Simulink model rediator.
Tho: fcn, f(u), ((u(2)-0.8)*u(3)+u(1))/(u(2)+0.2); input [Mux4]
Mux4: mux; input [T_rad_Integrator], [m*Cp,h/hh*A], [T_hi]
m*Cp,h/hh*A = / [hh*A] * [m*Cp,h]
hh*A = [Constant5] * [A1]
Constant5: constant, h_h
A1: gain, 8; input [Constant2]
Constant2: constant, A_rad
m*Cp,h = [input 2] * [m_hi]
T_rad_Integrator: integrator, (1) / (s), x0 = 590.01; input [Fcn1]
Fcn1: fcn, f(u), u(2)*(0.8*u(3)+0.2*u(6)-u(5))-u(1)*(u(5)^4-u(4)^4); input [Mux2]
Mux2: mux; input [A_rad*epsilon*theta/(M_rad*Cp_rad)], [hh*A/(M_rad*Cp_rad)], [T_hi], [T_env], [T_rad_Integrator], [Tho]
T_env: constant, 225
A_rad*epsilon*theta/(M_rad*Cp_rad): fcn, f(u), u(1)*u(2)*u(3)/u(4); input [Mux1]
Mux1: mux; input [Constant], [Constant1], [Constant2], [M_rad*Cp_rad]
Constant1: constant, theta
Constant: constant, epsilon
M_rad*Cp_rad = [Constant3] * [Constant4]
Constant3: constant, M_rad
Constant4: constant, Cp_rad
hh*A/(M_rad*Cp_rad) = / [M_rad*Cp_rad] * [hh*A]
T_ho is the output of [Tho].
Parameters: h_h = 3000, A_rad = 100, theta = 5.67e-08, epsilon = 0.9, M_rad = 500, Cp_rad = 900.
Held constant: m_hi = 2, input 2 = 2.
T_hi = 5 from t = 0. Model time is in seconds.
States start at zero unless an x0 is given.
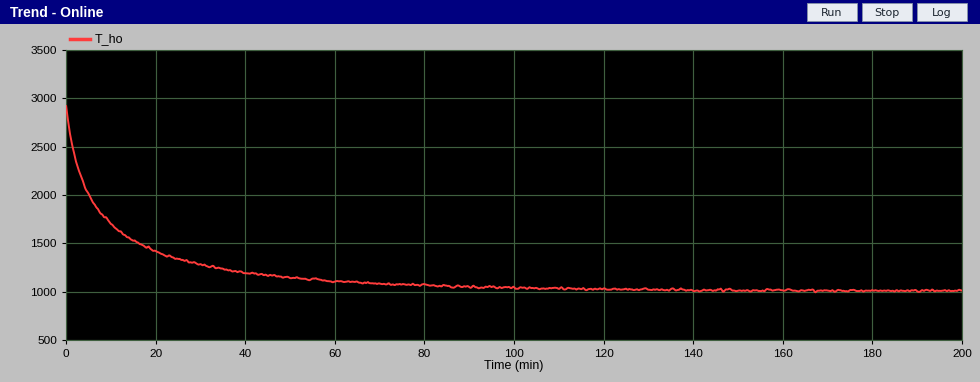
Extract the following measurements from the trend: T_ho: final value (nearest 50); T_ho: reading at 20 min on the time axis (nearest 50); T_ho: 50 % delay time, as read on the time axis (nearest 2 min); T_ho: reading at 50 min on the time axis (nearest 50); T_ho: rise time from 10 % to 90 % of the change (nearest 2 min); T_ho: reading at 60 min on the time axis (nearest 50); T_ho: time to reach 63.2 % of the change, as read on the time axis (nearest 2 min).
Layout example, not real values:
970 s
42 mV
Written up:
1000
1400
6 min
1150
40 min
1100
10 min
